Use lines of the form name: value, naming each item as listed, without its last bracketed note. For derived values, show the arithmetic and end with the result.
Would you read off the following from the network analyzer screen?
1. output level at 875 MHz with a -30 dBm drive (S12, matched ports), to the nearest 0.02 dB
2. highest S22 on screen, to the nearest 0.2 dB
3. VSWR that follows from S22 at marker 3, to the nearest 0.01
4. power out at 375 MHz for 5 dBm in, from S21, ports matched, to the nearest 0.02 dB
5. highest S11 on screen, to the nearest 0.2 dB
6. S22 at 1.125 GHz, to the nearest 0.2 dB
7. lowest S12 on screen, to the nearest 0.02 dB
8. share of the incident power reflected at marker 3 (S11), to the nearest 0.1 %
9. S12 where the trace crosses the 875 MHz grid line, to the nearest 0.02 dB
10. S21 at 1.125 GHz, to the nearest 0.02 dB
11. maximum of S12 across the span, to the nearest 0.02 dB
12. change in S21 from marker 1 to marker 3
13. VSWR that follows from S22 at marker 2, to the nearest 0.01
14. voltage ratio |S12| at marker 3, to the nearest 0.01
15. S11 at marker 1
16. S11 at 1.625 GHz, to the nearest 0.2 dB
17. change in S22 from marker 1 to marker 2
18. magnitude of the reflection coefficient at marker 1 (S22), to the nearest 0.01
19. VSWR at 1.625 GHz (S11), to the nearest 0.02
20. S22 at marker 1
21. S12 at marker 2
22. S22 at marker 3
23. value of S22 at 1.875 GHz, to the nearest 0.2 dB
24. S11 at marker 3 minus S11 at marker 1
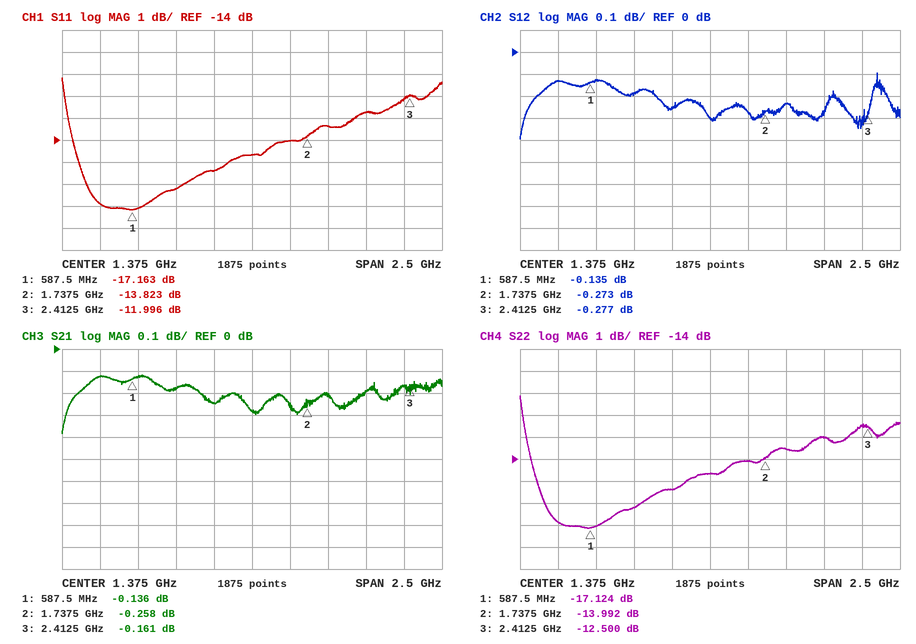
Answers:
output level at 875 MHz with a -30 dBm drive (S12, matched ports), to the nearest 0.02 dB: -30 dBm + (-0.18 dB) = -30.18 dBm
highest S22 on screen, to the nearest 0.2 dB: -11.2 dB
VSWR that follows from S22 at marker 3, to the nearest 0.01: (1 + 0.2371)/(1 − 0.2371) ≈ 1.62
power out at 375 MHz for 5 dBm in, from S21, ports matched, to the nearest 0.02 dB: 5 dBm + (-0.12 dB) = 4.88 dBm
highest S11 on screen, to the nearest 0.2 dB: -11.2 dB
S22 at 1.125 GHz, to the nearest 0.2 dB: -15.4 dB
lowest S12 on screen, to the nearest 0.02 dB: -0.40 dB
share of the incident power reflected at marker 3 (S11), to the nearest 0.1 %: 10^(-11.996/10) ≈ 6.3 %
S12 where the trace crosses the 875 MHz grid line, to the nearest 0.02 dB: -0.18 dB
S21 at 1.125 GHz, to the nearest 0.02 dB: -0.24 dB
maximum of S12 across the span, to the nearest 0.02 dB: -0.10 dB
change in S21 from marker 1 to marker 3: -0.161 − (-0.136) = -0.025 dB
VSWR that follows from S22 at marker 2, to the nearest 0.01: (1 + 0.1997)/(1 − 0.1997) ≈ 1.50
voltage ratio |S12| at marker 3, to the nearest 0.01: 10^(-0.277/20) ≈ 0.97
S11 at marker 1: -17.163 dB
S11 at 1.625 GHz, to the nearest 0.2 dB: -14.0 dB
change in S22 from marker 1 to marker 2: -13.992 − (-17.124) = 3.132 dB
magnitude of the reflection coefficient at marker 1 (S22), to the nearest 0.01: 10^(-17.124/20) ≈ 0.14
VSWR at 1.625 GHz (S11), to the nearest 0.02: |Γ| = 10^(-14/20) = 0.1995; VSWR = (1 + 0.1995)/(1 − 0.1995) ≈ 1.50
S22 at marker 1: -17.124 dB
S12 at marker 2: -0.273 dB
S22 at marker 3: -12.500 dB
value of S22 at 1.875 GHz, to the nearest 0.2 dB: -13.6 dB
S11 at marker 3 minus S11 at marker 1: -11.996 − (-17.163) = 5.167 dB
